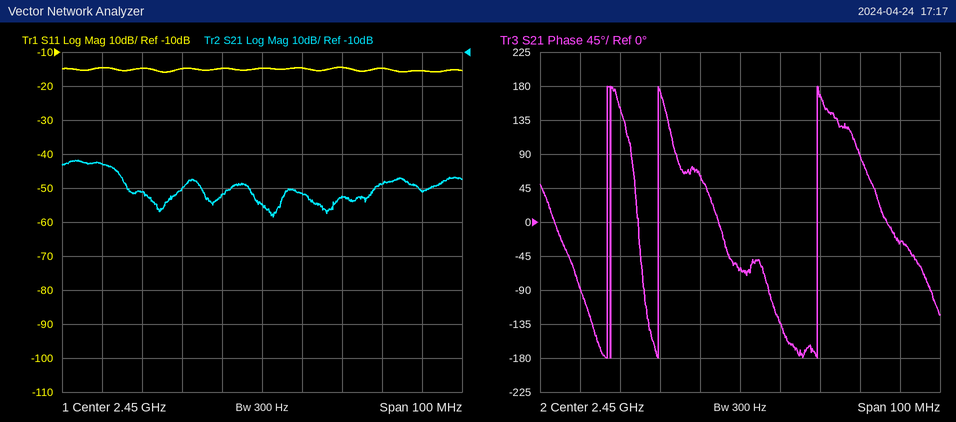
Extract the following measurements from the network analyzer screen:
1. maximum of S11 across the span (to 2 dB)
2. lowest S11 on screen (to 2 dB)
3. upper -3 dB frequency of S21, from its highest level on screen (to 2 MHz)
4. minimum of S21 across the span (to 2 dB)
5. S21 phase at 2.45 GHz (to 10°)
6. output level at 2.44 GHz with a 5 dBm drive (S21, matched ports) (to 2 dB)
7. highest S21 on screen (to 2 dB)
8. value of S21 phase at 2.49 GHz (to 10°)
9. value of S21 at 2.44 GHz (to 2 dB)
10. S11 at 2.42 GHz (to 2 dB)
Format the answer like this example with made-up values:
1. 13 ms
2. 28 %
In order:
1. -14 dB
2. -16 dB
3. 2.414 GHz
4. -58 dB
5. -60°
6. -46 dBm
7. -42 dB
8. -30°
9. -52 dB
10. -14 dB
